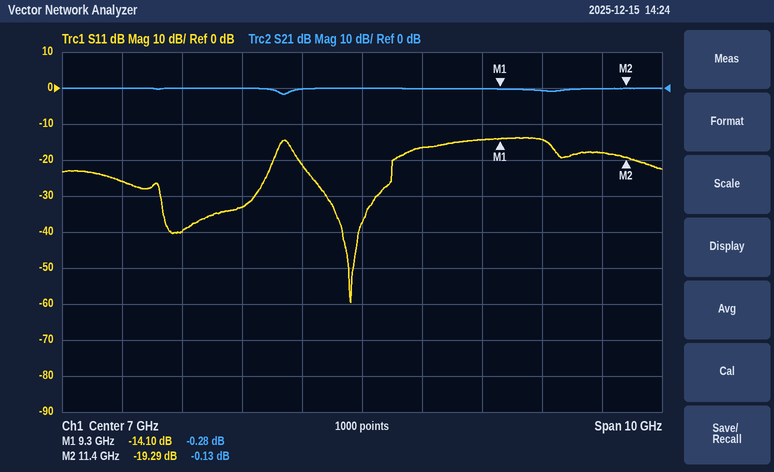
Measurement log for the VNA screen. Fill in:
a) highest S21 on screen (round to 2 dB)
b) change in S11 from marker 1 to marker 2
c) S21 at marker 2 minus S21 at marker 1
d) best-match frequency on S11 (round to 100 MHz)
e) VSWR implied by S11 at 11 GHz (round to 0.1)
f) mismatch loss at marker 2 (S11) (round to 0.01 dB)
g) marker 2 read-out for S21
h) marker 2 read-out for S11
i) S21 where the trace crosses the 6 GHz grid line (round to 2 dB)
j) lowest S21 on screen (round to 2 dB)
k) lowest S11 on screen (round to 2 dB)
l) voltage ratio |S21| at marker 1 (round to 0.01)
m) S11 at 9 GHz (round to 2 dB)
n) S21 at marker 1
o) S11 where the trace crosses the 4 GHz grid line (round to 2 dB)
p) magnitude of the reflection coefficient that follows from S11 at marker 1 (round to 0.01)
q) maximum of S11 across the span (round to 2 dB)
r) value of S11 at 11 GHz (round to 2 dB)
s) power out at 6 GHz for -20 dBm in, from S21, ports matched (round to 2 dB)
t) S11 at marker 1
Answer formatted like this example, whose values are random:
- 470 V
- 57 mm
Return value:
- 0 dB
- -5.19 dB
- 0.15 dB
- 6.8 GHz
- 1.3
- 0.05 dB
- -0.13 dB
- -19.29 dB
- 0 dB
- -2 dB
- -60 dB
- 0.97
- -14 dB
- -0.28 dB
- -40 dB
- 0.20
- -14 dB
- -18 dB
- -20 dBm
- -14.10 dB
